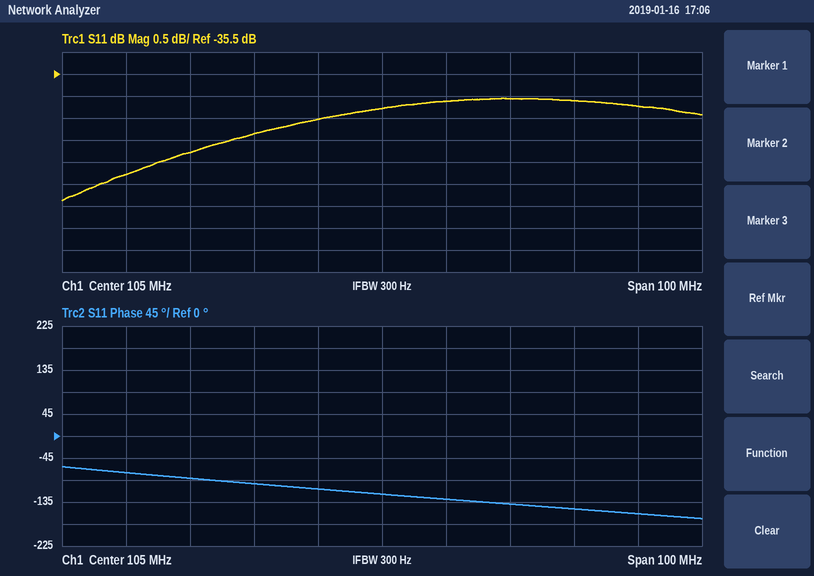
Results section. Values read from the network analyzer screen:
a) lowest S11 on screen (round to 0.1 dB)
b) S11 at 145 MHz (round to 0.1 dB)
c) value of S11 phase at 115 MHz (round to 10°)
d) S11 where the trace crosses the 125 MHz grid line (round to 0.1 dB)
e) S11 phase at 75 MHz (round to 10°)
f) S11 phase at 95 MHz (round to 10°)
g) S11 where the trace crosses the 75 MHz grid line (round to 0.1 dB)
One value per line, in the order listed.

-38.4 dB
-36.2 dB
-130°
-36.1 dB
-90°
-110°
-37.3 dB
